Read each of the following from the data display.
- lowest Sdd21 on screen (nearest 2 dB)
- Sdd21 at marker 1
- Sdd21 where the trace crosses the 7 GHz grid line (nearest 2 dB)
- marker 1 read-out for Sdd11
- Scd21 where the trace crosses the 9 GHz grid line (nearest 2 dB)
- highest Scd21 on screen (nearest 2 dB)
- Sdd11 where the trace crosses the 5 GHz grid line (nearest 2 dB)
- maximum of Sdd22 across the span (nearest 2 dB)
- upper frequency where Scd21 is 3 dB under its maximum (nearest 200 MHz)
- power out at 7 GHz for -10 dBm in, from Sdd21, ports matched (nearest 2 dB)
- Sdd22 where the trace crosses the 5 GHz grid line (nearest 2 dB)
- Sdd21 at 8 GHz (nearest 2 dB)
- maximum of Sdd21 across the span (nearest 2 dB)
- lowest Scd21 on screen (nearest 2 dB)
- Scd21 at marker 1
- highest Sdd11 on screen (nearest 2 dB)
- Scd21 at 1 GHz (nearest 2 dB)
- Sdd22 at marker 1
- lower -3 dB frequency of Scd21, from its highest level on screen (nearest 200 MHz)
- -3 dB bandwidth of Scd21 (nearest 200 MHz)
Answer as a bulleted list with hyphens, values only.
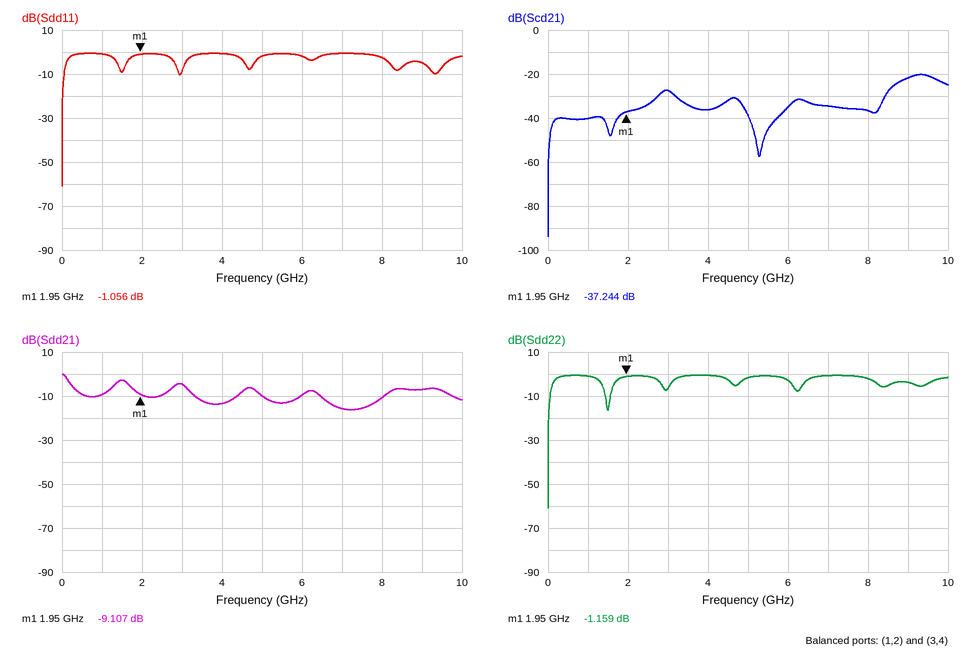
- -16 dB
- -9.107 dB
- -16 dB
- -1.056 dB
- -22 dB
- -20 dB
- -2 dB
- 0 dB
- 9.8 GHz
- -26 dBm
- -2 dB
- -10 dB
- 0 dB
- -94 dB
- -37.244 dB
- 0 dB
- -40 dB
- -1.159 dB
- 8.8 GHz
- 1.0 GHz
